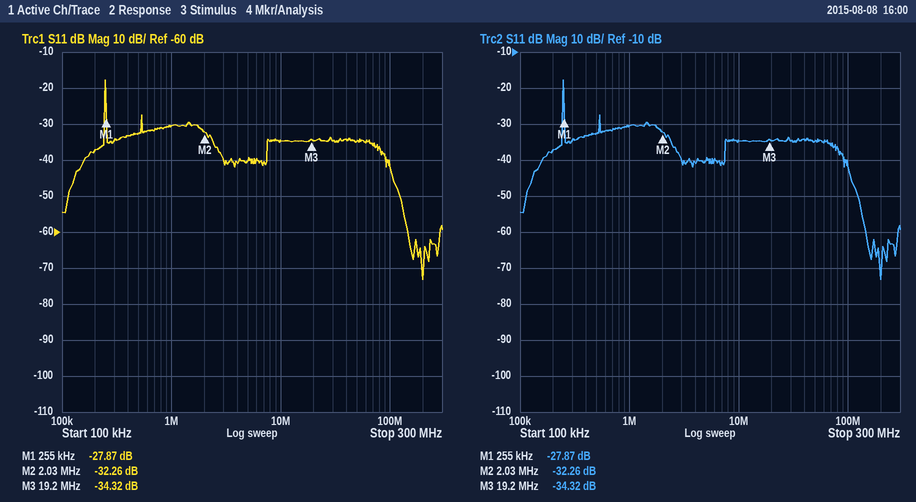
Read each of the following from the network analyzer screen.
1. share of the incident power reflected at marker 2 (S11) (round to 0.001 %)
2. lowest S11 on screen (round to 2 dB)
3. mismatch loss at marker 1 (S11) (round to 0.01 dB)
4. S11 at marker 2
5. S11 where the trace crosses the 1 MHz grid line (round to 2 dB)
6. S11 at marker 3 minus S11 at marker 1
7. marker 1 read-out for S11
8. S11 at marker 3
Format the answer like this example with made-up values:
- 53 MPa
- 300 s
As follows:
- 0.059 %
- -74 dB
- 0.01 dB
- -32.26 dB
- -30 dB
- -6.45 dB
- -27.87 dB
- -34.32 dB
